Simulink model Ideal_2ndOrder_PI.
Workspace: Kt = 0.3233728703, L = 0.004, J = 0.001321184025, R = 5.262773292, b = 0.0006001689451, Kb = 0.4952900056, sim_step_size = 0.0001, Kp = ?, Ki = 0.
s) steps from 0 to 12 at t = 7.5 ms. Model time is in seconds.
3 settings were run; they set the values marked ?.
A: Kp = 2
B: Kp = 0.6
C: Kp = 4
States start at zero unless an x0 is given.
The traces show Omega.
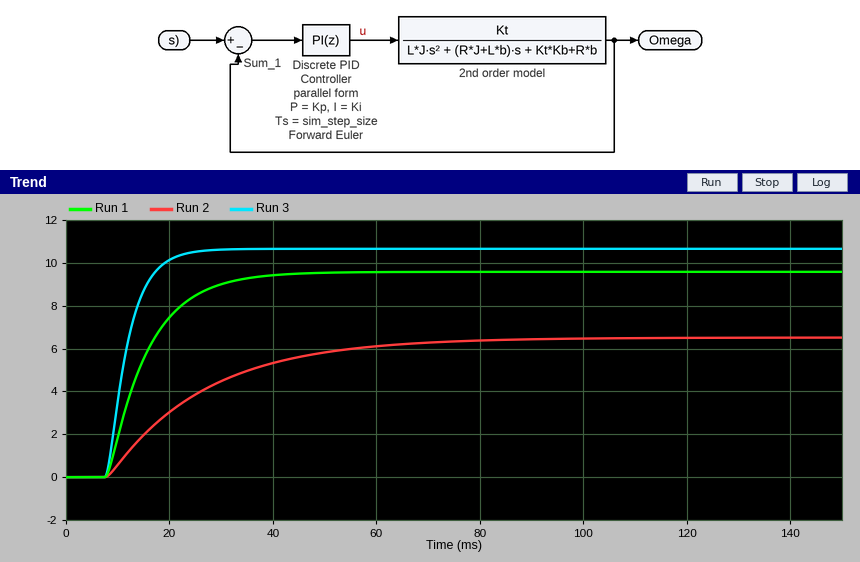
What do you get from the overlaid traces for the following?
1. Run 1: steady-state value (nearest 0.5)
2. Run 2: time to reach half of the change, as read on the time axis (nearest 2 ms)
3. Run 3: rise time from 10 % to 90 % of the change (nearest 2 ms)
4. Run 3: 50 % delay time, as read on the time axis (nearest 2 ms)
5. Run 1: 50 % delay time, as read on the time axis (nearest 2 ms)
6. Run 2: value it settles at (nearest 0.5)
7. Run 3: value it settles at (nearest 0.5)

9.5
22 ms
8 ms
12 ms
14 ms
6.5
10.5
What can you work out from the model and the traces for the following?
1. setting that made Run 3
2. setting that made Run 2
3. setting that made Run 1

C
B
A
